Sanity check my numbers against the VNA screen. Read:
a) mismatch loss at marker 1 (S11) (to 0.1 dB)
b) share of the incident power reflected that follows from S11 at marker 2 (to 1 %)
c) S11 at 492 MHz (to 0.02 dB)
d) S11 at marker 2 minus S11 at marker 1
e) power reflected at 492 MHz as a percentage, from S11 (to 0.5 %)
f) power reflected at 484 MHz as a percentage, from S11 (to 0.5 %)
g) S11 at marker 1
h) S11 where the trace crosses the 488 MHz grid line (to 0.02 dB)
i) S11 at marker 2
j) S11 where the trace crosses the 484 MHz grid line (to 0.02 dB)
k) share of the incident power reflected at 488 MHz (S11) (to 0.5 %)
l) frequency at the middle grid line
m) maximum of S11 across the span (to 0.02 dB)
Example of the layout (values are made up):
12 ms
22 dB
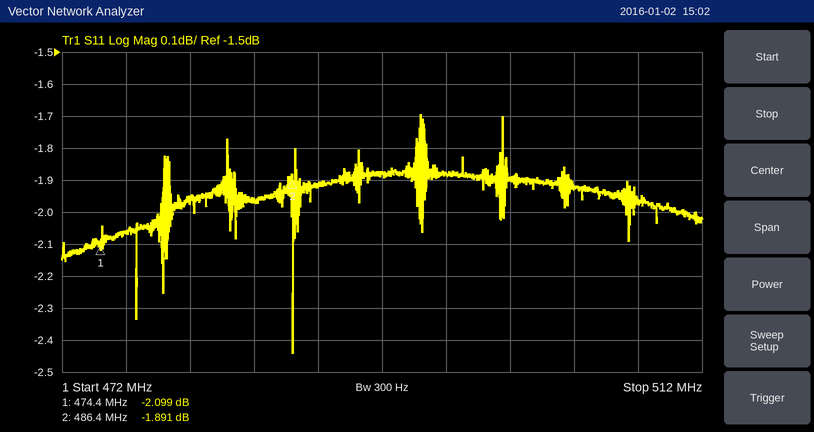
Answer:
4.2 dB
65 %
-1.88 dB
0.208 dB
65.0 %
63.5 %
-2.099 dB
-1.92 dB
-1.891 dB
-1.96 dB
64.5 %
492 MHz
-1.70 dB
